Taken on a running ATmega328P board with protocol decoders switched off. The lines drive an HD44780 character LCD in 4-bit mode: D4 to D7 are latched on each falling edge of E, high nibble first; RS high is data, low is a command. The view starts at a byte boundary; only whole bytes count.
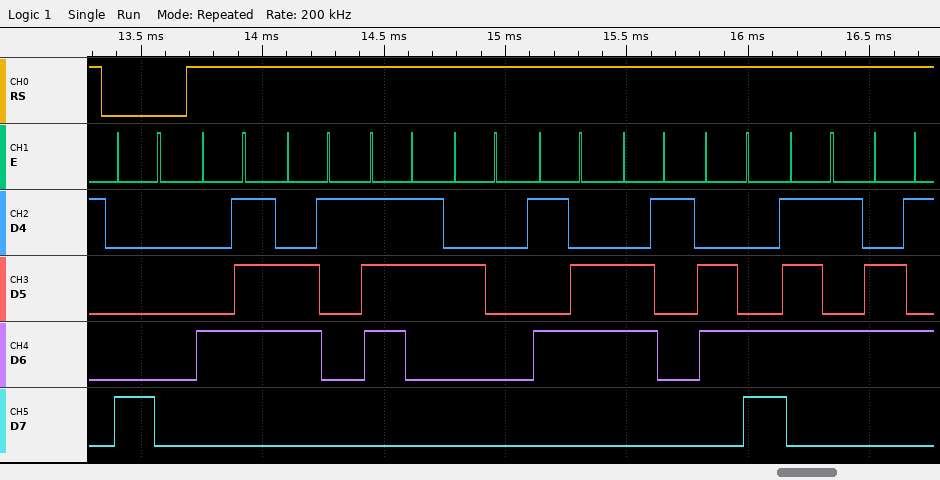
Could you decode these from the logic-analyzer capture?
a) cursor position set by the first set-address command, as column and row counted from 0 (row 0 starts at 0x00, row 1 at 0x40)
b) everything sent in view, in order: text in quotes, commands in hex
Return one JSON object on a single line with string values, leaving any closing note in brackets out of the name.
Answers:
{"cursor position set by the first set-address command, as column and row counted from 0": "column 0, row 0", "everything sent in view, in order: text in quotes, commands in hex": "0x80 \"Gas Value\""}
